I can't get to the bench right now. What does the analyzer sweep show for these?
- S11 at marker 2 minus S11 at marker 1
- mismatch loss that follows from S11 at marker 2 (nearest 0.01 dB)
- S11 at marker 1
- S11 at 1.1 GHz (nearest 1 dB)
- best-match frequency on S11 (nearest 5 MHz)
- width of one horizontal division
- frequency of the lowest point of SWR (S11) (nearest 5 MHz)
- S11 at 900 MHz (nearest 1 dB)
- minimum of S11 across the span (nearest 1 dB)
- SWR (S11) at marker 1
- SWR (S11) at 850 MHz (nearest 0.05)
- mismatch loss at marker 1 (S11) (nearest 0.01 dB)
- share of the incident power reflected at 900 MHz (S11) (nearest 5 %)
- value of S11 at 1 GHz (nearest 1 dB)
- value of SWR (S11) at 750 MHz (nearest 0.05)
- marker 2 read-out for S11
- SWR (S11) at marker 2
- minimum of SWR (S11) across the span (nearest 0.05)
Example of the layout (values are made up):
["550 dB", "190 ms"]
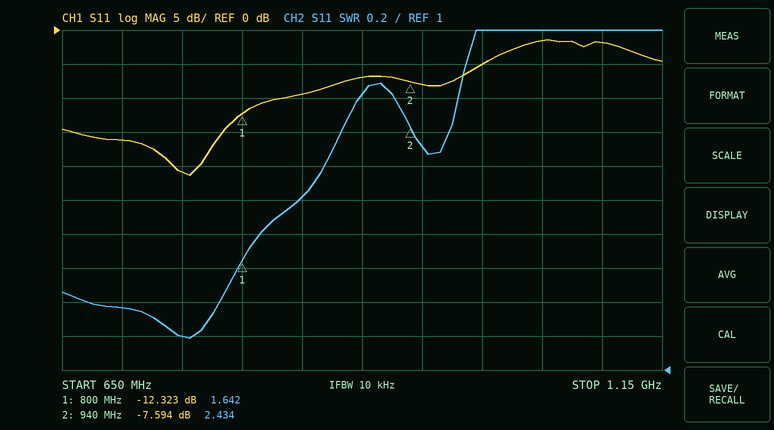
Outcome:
["4.729 dB", "0.83 dB", "-12.323 dB", "-2 dB", "755 MHz", "50 MHz", "755 MHz", "-7 dB", "-21 dB", "1.642", "2.00", "0.26 dB", "20 %", "-5 dB", "1.20", "-7.594 dB", "2.434", "1.20"]
